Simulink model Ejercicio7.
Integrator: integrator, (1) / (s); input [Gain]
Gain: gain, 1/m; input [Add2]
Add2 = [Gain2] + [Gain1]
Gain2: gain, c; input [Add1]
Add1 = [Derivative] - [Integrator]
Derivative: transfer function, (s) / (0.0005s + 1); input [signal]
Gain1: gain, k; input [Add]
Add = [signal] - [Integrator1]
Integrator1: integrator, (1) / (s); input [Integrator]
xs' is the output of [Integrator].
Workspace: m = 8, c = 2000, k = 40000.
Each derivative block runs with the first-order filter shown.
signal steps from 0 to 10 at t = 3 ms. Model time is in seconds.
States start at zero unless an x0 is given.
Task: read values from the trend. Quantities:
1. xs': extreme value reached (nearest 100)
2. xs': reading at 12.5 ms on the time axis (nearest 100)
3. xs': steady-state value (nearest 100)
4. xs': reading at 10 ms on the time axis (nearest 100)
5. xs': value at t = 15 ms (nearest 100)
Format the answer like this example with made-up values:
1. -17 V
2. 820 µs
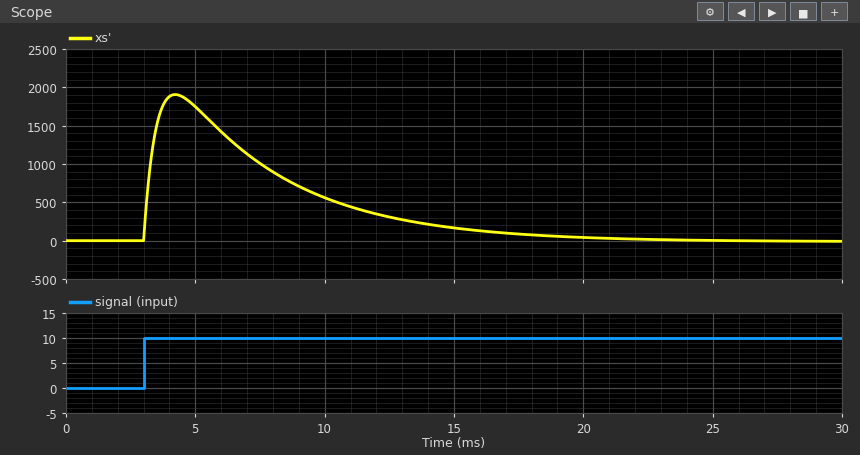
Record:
1. 1900
2. 300
3. 0
4. 600
5. 200
